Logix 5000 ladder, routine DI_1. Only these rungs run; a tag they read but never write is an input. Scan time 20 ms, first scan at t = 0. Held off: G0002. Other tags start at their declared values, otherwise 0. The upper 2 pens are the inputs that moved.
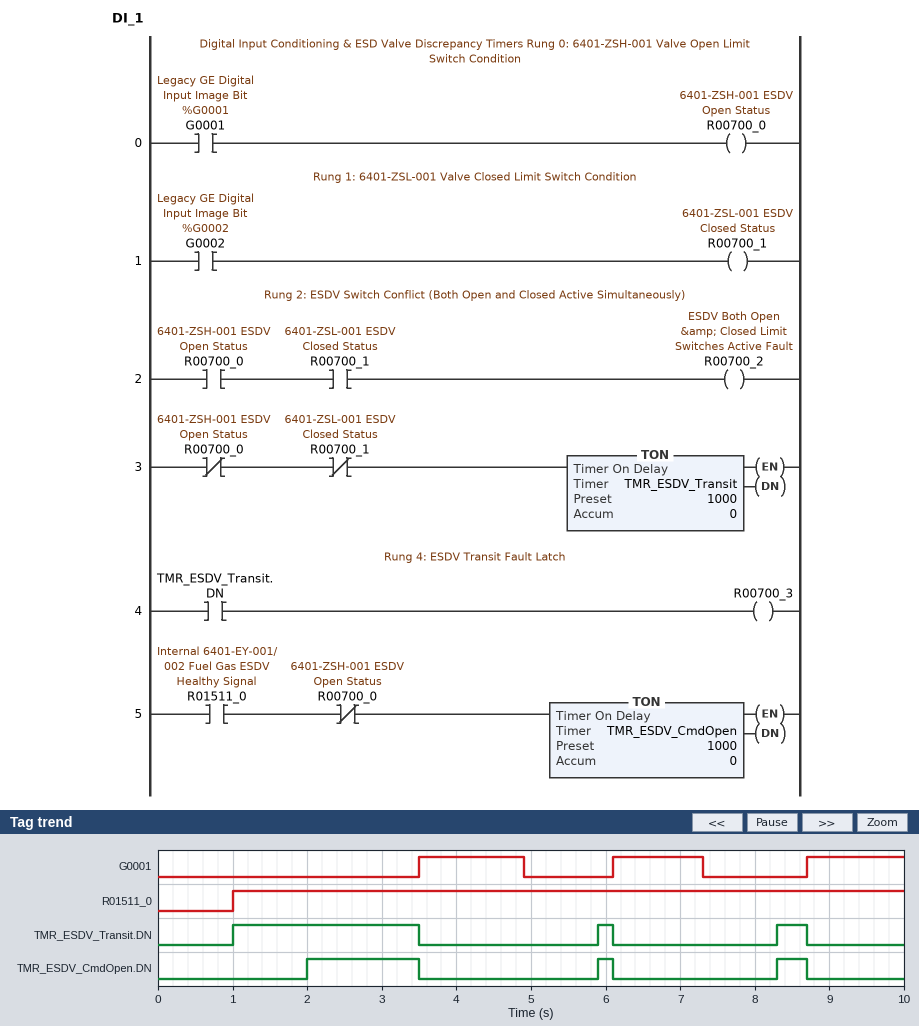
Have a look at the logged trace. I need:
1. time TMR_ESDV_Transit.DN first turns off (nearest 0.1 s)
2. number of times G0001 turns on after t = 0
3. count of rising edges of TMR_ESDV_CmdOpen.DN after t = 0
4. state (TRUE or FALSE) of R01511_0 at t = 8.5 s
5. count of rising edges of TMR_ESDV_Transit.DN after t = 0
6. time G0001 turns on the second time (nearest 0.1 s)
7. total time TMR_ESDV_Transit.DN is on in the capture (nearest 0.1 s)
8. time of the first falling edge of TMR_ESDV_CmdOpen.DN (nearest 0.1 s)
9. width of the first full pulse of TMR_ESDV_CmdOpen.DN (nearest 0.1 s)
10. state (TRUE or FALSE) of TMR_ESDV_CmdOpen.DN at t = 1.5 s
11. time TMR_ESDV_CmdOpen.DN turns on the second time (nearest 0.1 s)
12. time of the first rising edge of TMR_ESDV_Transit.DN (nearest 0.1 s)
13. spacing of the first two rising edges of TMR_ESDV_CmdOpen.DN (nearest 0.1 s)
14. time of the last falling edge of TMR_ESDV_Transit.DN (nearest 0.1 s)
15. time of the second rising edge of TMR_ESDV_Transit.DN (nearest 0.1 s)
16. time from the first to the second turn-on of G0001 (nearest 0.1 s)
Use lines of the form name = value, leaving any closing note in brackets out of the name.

time TMR_ESDV_Transit.DN first turns off = 3.5 s
number of times G0001 turns on after t = 0 = 3
count of rising edges of TMR_ESDV_CmdOpen.DN after t = 0 = 3
state (TRUE or FALSE) of R01511_0 at t = 8.5 s = TRUE
count of rising edges of TMR_ESDV_Transit.DN after t = 0 = 3
time G0001 turns on the second time = 6.1 s
total time TMR_ESDV_Transit.DN is on in the capture = 3.1 s
time of the first falling edge of TMR_ESDV_CmdOpen.DN = 3.5 s
width of the first full pulse of TMR_ESDV_CmdOpen.DN = 1.5 s
state (TRUE or FALSE) of TMR_ESDV_CmdOpen.DN at t = 1.5 s = FALSE
time TMR_ESDV_CmdOpen.DN turns on the second time = 5.9 s
time of the first rising edge of TMR_ESDV_Transit.DN = 1.0 s
spacing of the first two rising edges of TMR_ESDV_CmdOpen.DN = 3.9 s
time of the last falling edge of TMR_ESDV_Transit.DN = 8.7 s
time of the second rising edge of TMR_ESDV_Transit.DN = 5.9 s
time from the first to the second turn-on of G0001 = 2.6 s
